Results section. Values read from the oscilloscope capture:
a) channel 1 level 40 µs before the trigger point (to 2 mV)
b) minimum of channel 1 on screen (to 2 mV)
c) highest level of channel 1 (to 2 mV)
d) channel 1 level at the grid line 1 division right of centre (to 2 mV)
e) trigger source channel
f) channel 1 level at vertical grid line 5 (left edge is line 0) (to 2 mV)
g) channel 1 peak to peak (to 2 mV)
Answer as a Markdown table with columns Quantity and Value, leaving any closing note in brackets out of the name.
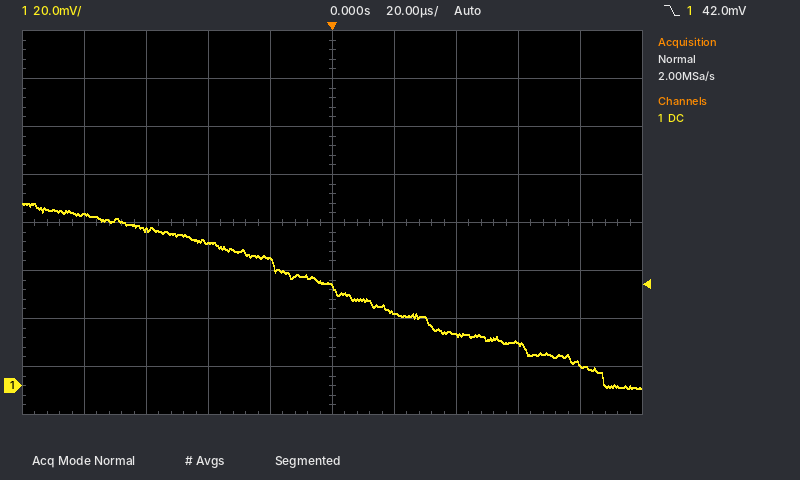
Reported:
| Quantity | Value |
|---|---|
| channel 1 level 40 µs before the trigger point | 60 mV |
| minimum of channel 1 on screen | -2 mV |
| highest level of channel 1 | 76 mV |
| channel 1 level at the grid line 1 division right of centre | 30 mV |
| trigger source channel | channel 1 |
| channel 1 level at vertical grid line 5 (left edge is line 0) | 42 mV |
| channel 1 peak to peak | 78 mV |
